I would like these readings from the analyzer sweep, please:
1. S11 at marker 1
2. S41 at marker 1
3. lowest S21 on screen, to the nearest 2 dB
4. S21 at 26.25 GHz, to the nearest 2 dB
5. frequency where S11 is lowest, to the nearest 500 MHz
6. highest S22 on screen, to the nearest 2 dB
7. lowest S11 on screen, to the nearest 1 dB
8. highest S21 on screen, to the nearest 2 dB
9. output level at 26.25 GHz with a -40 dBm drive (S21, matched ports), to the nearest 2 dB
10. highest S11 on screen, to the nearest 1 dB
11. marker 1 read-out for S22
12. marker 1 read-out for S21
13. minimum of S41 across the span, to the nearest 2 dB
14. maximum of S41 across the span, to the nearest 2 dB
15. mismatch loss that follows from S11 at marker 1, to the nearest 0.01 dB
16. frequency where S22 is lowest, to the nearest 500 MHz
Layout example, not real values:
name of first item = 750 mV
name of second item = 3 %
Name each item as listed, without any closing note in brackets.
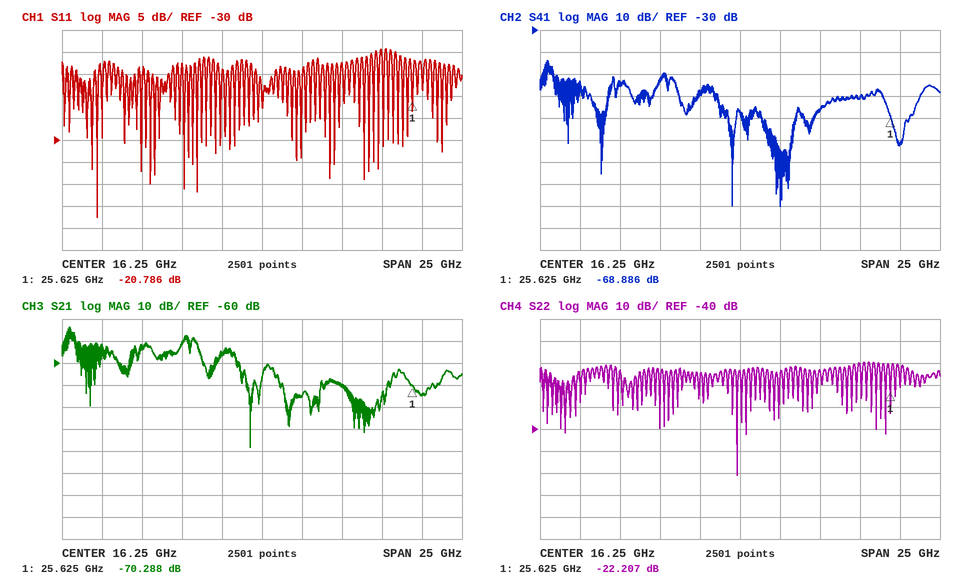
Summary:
S11 at marker 1 = -20.786 dB
S41 at marker 1 = -68.886 dB
lowest S21 on screen, to the nearest 2 dB = -98 dB
S21 at 26.25 GHz, to the nearest 2 dB = -74 dB
frequency where S11 is lowest, to the nearest 500 MHz = 6.0 GHz
highest S22 on screen, to the nearest 2 dB = -10 dB
lowest S11 on screen, to the nearest 1 dB = -48 dB
highest S21 on screen, to the nearest 2 dB = -44 dB
output level at 26.25 GHz with a -40 dBm drive (S21, matched ports), to the nearest 2 dB = -114 dBm
highest S11 on screen, to the nearest 1 dB = -9 dB
marker 1 read-out for S22 = -22.207 dB
marker 1 read-out for S21 = -70.288 dB
minimum of S41 across the span, to the nearest 2 dB = -110 dB
maximum of S41 across the span, to the nearest 2 dB = -44 dB
mismatch loss that follows from S11 at marker 1, to the nearest 0.01 dB = 0.04 dB
frequency where S22 is lowest, to the nearest 500 MHz = 16.0 GHz
